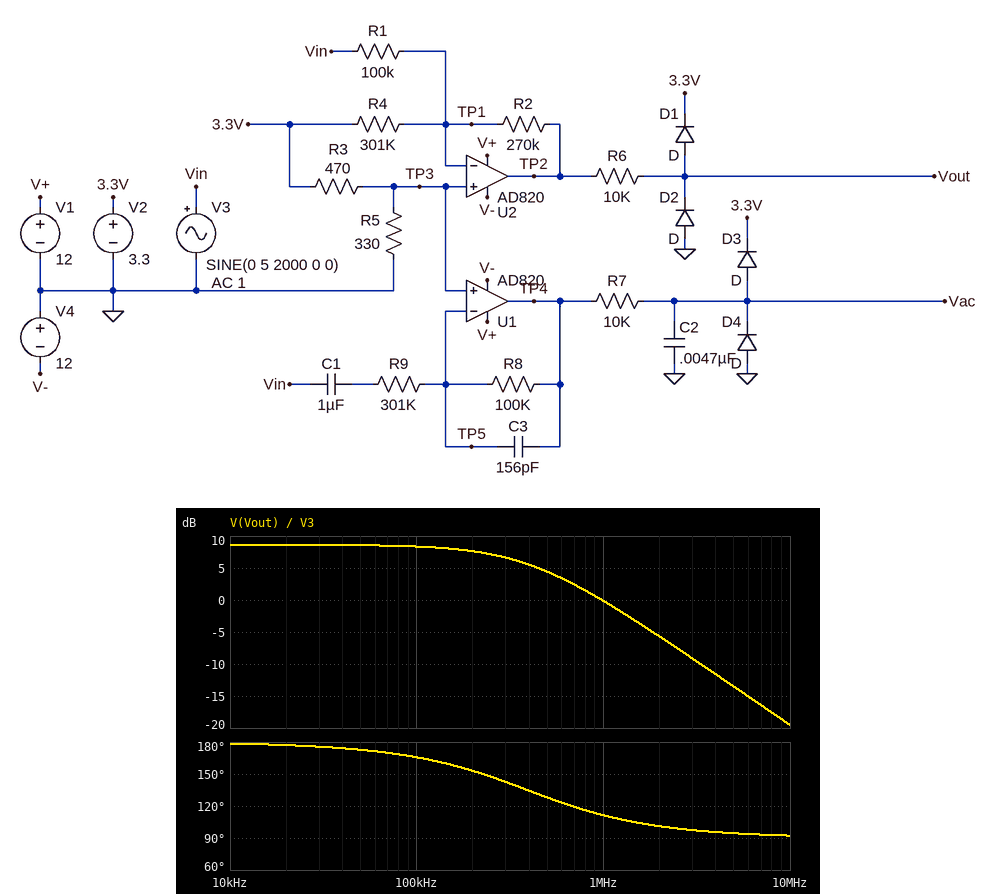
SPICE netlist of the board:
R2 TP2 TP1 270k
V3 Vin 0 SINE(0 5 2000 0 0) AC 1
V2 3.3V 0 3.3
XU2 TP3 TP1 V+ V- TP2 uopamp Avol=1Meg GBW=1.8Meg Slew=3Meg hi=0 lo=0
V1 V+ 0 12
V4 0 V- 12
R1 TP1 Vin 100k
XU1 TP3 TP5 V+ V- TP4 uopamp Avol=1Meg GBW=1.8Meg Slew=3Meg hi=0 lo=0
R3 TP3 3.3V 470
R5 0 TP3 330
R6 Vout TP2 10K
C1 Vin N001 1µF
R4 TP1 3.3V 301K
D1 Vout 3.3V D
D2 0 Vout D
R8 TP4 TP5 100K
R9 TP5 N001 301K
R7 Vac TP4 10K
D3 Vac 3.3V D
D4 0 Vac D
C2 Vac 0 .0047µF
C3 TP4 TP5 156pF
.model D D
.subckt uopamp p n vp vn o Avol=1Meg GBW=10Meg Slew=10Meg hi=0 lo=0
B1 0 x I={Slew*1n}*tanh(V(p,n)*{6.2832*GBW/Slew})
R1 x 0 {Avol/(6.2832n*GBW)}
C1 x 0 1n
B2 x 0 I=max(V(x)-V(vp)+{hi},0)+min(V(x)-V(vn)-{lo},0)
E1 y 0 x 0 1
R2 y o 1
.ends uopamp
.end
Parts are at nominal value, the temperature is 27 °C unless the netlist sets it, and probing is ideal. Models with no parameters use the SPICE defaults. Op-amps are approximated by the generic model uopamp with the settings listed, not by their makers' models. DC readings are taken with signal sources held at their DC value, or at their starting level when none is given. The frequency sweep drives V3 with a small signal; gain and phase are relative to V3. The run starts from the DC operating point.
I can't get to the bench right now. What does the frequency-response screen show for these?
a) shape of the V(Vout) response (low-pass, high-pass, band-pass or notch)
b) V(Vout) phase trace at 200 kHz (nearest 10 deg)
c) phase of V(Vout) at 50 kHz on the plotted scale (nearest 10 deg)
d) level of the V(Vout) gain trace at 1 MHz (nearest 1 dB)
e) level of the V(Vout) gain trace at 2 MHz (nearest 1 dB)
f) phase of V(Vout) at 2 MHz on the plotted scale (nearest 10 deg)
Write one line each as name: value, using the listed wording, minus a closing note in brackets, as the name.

shape of the V(Vout) response: low-pass
V(Vout) phase trace at 200 kHz: 150 deg
phase of V(Vout) at 50 kHz on the plotted scale: 170 deg
level of the V(Vout) gain trace at 1 MHz: 0 dB
level of the V(Vout) gain trace at 2 MHz: -6 dB
phase of V(Vout) at 2 MHz on the plotted scale: 100 deg
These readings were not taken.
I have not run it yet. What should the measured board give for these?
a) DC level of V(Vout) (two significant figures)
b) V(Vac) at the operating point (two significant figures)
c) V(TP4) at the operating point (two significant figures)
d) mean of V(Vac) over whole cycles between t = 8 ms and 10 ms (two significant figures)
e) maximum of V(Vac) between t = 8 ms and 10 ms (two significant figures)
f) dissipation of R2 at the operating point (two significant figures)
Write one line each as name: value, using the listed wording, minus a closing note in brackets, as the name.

DC level of V(Vout): 3.3 V
V(Vac) at the operating point: 1.4 V
V(TP4) at the operating point: 1.4 V
mean of V(Vac) over whole cycles between t = 8 ms and 10 ms: 1.4 V
maximum of V(Vac) between t = 8 ms and 10 ms: 2.8 V
dissipation of R2 at the operating point: 14 µW
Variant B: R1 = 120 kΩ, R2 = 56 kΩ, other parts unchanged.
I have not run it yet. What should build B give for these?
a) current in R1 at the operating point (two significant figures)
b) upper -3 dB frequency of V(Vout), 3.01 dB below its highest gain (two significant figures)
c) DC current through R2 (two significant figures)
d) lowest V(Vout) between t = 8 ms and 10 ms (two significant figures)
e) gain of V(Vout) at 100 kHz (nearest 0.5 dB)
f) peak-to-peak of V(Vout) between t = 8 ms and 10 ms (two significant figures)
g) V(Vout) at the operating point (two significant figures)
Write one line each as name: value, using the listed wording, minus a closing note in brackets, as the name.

current in R1 at the operating point: 11 µA
upper -3 dB frequency of V(Vout), 3.01 dB below its highest gain: 1.1 MHz
DC current through R2: 4.9 µA
lowest V(Vout) between t = 8 ms and 10 ms: -550 mV
gain of V(Vout) at 100 kHz: -6.5 dB
peak-to-peak of V(Vout) between t = 8 ms and 10 ms: 4.4 V
V(Vout) at the operating point: 1.6 V
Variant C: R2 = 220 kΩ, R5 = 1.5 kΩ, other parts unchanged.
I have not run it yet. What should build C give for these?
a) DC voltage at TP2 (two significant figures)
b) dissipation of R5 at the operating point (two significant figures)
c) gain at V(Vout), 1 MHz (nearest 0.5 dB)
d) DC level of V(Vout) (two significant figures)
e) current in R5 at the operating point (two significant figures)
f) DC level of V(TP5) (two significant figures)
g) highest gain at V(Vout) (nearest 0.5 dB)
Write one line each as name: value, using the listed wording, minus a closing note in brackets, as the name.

DC voltage at TP2: 7.5 V
dissipation of R5 at the operating point: 4.2 mW
gain at V(Vout), 1 MHz: -43.5 dB
DC level of V(Vout): 3.9 V
current in R5 at the operating point: 1.7 mA
DC level of V(TP5): 2.5 V
highest gain at V(Vout): -36.0 dB
